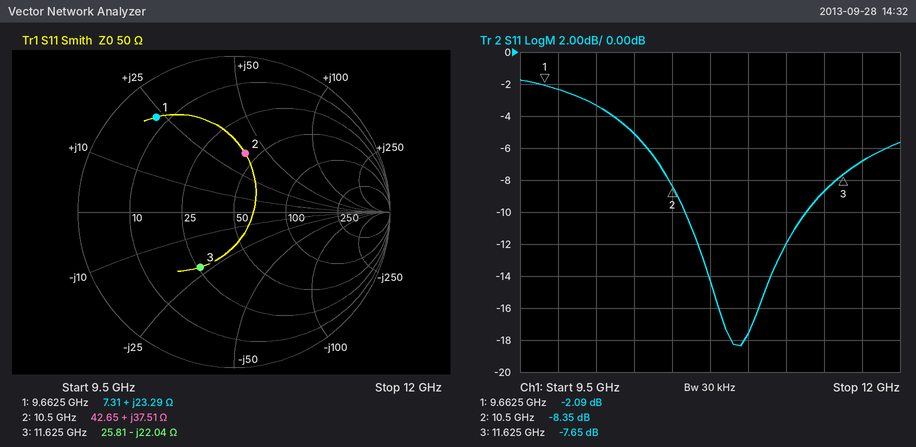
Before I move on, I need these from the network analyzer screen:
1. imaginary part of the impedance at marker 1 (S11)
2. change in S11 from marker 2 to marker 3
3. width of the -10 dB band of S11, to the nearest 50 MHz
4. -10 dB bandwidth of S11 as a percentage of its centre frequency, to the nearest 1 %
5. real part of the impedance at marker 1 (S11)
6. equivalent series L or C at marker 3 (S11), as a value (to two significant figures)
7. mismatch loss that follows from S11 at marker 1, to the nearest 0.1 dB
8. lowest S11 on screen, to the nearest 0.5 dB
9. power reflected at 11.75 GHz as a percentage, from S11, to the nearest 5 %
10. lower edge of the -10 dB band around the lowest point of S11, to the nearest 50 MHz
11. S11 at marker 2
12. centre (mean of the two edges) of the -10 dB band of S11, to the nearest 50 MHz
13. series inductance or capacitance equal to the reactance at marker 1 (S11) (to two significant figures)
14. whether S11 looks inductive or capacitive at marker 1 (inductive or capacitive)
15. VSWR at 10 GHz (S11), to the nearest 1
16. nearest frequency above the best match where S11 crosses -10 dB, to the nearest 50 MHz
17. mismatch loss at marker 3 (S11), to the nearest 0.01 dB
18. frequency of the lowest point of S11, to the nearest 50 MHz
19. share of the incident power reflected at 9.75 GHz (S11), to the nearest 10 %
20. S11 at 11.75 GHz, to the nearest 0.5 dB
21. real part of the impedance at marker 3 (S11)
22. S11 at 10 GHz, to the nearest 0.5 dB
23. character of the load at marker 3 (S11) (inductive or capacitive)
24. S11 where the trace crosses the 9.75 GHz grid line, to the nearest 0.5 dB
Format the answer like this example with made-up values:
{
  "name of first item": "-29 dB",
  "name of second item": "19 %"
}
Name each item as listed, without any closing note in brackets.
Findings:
{
  "imaginary part of the impedance at marker 1": "+23.29 Ω",
  "change in S11 from marker 2 to marker 3": "0.70 dB",
  "width of the -10 dB band of S11, to the nearest 50 MHz": "800 MHz",
  "-10 dB bandwidth of S11 as a percentage of its centre frequency, to the nearest 1 %": "7 %",
  "real part of the impedance at marker 1": "7.31 Ω",
  "equivalent series L or C at marker 3 (S11), as a value": "620 fF",
  "mismatch loss that follows from S11 at marker 1, to the nearest 0.1 dB": "4.2 dB",
  "lowest S11 on screen, to the nearest 0.5 dB": "-18.5 dB",
  "power reflected at 11.75 GHz as a percentage, from S11, to the nearest 5 %": "20 %",
  "lower edge of the -10 dB band around the lowest point of S11, to the nearest 50 MHz": "10.60 GHz",
  "S11 at marker 2": "-8.35 dB",
  "centre (mean of the two edges) of the -10 dB band of S11, to the nearest 50 MHz": "11.00 GHz",
  "series inductance or capacitance equal to the reactance at marker 1 (S11)": "380 pH",
  "whether S11 looks inductive or capacitive at marker 1": "inductive",
  "VSWR at 10 GHz (S11), to the nearest 1": "5",
  "nearest frequency above the best match where S11 crosses -10 dB, to the nearest 50 MHz": "11.40 GHz",
  "mismatch loss at marker 3 (S11), to the nearest 0.01 dB": "0.82 dB",
  "frequency of the lowest point of S11, to the nearest 50 MHz": "10.95 GHz",
  "share of the incident power reflected at 9.75 GHz (S11), to the nearest 10 %": "60 %",
  "S11 at 11.75 GHz, to the nearest 0.5 dB": "-7.0 dB",
  "real part of the impedance at marker 3": "25.81 Ω",
  "S11 at 10 GHz, to the nearest 0.5 dB": "-3.5 dB",
  "character of the load at marker 3 (S11)": "capacitive",
  "S11 where the trace crosses the 9.75 GHz grid line, to the nearest 0.5 dB": "-2.5 dB"
}
